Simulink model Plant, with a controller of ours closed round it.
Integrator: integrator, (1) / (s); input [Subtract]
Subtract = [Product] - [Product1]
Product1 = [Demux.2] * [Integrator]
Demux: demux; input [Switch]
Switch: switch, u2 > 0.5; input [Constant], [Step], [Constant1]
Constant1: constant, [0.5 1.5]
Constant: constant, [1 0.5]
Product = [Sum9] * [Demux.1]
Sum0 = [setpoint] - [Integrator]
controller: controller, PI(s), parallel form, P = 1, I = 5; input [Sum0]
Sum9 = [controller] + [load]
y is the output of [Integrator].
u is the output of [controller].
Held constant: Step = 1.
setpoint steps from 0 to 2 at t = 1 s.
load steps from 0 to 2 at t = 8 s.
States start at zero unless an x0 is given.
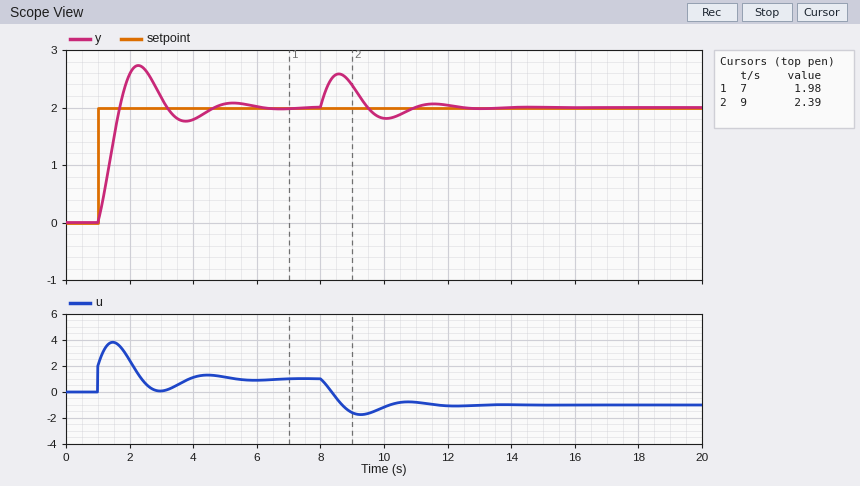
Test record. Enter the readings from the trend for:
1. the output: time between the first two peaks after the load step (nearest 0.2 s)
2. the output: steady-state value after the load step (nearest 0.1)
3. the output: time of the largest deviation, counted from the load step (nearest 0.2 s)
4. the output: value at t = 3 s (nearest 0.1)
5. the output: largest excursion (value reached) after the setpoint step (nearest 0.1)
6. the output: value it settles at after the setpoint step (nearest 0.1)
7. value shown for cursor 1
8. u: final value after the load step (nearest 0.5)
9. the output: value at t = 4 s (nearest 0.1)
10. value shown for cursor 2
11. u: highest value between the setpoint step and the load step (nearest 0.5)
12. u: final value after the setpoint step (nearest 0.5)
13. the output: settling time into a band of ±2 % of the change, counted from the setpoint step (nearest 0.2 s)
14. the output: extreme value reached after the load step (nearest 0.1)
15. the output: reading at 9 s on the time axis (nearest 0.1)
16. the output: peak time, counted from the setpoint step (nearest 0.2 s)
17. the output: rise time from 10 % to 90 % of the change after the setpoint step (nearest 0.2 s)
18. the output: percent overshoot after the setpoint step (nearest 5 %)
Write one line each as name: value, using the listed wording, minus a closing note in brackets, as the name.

the output: time between the first two peaks after the load step: 3.0 s
the output: steady-state value after the load step: 2.0
the output: time of the largest deviation, counted from the load step: 0.6 s
the output: value at t = 3 s: 2.2
the output: largest excursion (value reached) after the setpoint step: 2.7
the output: value it settles at after the setpoint step: 2.0
value shown for cursor 1: 1.98
u: final value after the load step: -1.0
the output: value at t = 4 s: 1.8
value shown for cursor 2: 2.39
u: highest value between the setpoint step and the load step: 4.0
u: final value after the setpoint step: 1.0
the output: settling time into a band of ±2 % of the change, counted from the setpoint step: 4.8 s
the output: extreme value reached after the load step: 2.6
the output: reading at 9 s on the time axis: 2.4
the output: peak time, counted from the setpoint step: 1.2 s
the output: rise time from 10 % to 90 % of the change after the setpoint step: 0.6 s
the output: percent overshoot after the setpoint step: 35 %
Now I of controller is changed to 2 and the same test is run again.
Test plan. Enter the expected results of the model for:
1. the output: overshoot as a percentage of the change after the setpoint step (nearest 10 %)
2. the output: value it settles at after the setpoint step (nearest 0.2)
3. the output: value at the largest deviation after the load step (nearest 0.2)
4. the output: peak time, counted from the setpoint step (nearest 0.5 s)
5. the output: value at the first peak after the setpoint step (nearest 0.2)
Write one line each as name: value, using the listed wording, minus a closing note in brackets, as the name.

the output: overshoot as a percentage of the change after the setpoint step: 20 %
the output: value it settles at after the setpoint step: 2.0
the output: value at the largest deviation after the load step: 2.8
the output: peak time, counted from the setpoint step: 2.0 s
the output: value at the first peak after the setpoint step: 2.4
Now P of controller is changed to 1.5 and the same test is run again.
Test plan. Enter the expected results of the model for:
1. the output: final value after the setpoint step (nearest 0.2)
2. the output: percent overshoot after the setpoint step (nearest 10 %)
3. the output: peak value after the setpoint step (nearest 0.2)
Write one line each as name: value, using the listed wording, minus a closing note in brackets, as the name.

the output: final value after the setpoint step: 2.0
the output: percent overshoot after the setpoint step: 30 %
the output: peak value after the setpoint step: 2.6
